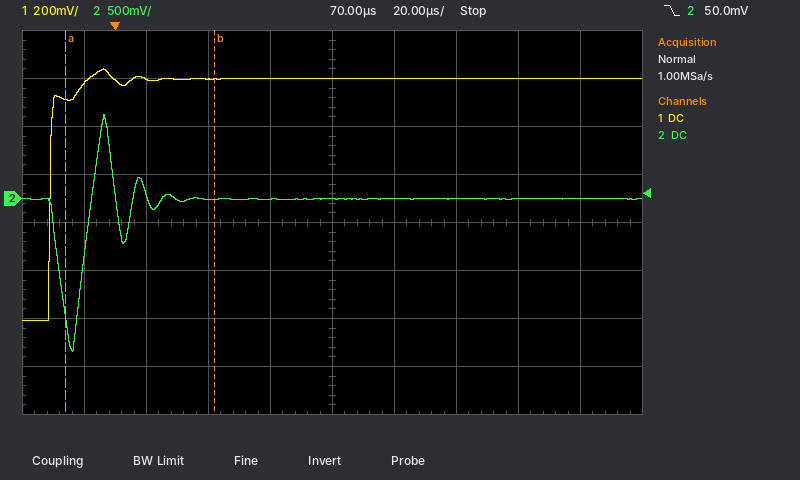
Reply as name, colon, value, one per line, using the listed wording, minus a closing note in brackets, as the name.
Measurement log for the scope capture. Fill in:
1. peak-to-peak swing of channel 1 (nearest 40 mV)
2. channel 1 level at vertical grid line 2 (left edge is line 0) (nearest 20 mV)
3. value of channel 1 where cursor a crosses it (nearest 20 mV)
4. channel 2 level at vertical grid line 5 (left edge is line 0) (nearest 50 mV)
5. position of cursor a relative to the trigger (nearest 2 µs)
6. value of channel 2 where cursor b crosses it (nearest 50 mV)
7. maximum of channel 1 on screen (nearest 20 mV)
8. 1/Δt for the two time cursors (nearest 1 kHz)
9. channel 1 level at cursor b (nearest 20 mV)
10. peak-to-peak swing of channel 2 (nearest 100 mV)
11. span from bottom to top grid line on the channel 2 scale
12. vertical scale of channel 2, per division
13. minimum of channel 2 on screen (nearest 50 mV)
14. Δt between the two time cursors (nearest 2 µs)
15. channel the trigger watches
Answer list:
peak-to-peak swing of channel 1: 1.04 V
channel 1 level at vertical grid line 2 (left edge is line 0): 500 mV
value of channel 1 where cursor a crosses it: 420 mV
channel 2 level at vertical grid line 5 (left edge is line 0): 0 mV
position of cursor a relative to the trigger: -16 µs
value of channel 2 where cursor b crosses it: 0 mV
maximum of channel 1 on screen: 540 mV
1/Δt for the two time cursors: 21 kHz
channel 1 level at cursor b: 500 mV
peak-to-peak swing of channel 2: 2.50 V
span from bottom to top grid line on the channel 2 scale: 4 V
vertical scale of channel 2, per division: 500 mV
minimum of channel 2 on screen: -1.60 V
Δt between the two time cursors: 48 µs
channel the trigger watches: channel 2
